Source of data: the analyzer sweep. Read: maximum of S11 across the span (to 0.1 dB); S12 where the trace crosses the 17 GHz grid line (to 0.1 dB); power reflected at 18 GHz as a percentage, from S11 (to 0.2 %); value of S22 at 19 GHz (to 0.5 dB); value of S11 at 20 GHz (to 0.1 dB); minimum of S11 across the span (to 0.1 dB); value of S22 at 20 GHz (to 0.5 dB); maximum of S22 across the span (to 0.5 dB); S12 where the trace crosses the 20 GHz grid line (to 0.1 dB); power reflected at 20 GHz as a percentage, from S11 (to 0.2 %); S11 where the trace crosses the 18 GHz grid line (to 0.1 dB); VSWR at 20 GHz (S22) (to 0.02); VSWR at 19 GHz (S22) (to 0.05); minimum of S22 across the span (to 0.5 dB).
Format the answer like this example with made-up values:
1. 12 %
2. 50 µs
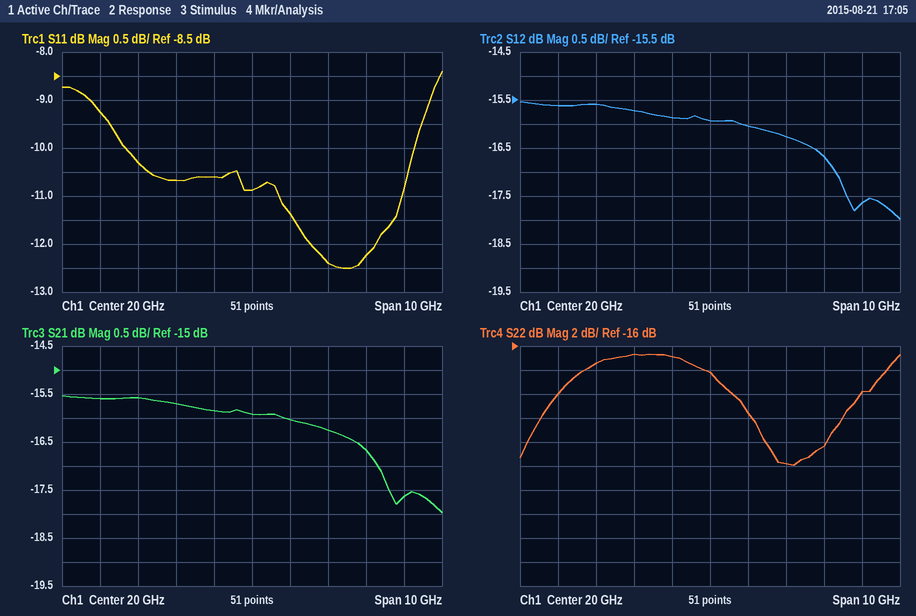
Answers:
1. -8.4 dB
2. -15.6 dB
3. 8.6 %
4. -17.0 dB
5. -10.9 dB
6. -12.5 dB
7. -18.0 dB
8. -16.5 dB
9. -15.9 dB
10. 8.2 %
11. -10.7 dB
12. 1.28
13. 1.35
14. -26.0 dB
